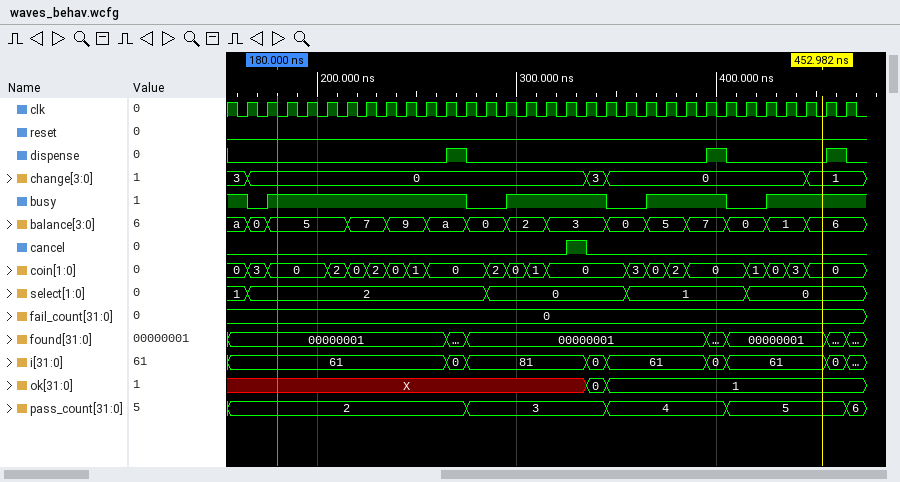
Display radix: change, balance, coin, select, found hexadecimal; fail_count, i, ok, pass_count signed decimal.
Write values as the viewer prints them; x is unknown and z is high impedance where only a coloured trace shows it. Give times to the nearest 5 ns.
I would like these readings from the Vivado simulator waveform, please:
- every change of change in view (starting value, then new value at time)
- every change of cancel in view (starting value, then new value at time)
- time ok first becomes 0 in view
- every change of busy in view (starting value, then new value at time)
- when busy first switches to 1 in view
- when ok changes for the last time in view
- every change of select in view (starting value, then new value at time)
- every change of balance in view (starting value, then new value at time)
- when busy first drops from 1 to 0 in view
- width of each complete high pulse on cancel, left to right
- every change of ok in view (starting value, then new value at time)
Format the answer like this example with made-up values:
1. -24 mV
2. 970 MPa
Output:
1. 3, 0 at 165 ns, 3 at 335 ns, 0 at 345 ns, 1 at 445 ns
2. 0, 1 at 325 ns, 0 at 335 ns
3. 335 ns
4. 1, 0 at 165 ns, 1 at 175 ns, 0 at 275 ns, 1 at 295 ns, 0 at 345 ns, 1 at 365 ns, 0 at 405 ns, 1 at 425 ns
5. 175 ns
6. 345 ns
7. 1, 2 at 165 ns, 0 at 285 ns, 1 at 355 ns, 0 at 415 ns
8. a, 0 at 165 ns, 5 at 175 ns, 7 at 215 ns, 9 at 235 ns, a at 255 ns, 0 at 275 ns, 2 at 295 ns, 3 at 315 ns, 0 at 345 ns, 5 at 365 ns, 7 at 385 ns, 0 at 405 ns, 1 at 425 ns, 6 at 445 ns
9. 165 ns
10. 10 ns
11. X, 0 at 335 ns, 1 at 345 ns
